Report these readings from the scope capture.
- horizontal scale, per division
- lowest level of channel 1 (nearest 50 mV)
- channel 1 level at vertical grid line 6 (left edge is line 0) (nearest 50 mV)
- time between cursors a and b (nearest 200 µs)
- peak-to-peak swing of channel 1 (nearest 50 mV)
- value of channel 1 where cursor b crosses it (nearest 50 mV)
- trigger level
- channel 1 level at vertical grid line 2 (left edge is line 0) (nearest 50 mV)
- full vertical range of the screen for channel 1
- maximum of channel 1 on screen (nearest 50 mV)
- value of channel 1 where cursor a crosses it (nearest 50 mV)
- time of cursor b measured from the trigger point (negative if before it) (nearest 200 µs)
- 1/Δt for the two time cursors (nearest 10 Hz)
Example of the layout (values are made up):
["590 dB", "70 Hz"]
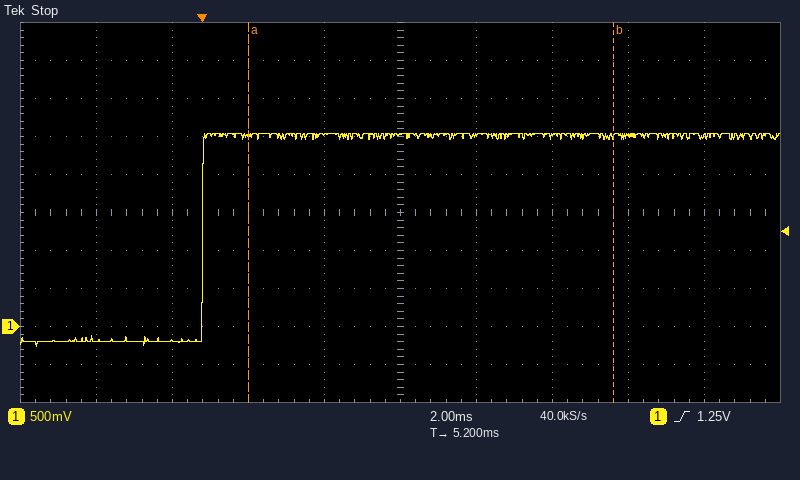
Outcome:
["2 ms", "-250 mV", "2.50 V", "9.6 ms", "2.80 V", "2.50 V", "1.25 V", "-200 mV", "5 V", "2.55 V", "2.50 V", "+10.8 ms", "100 Hz"]
